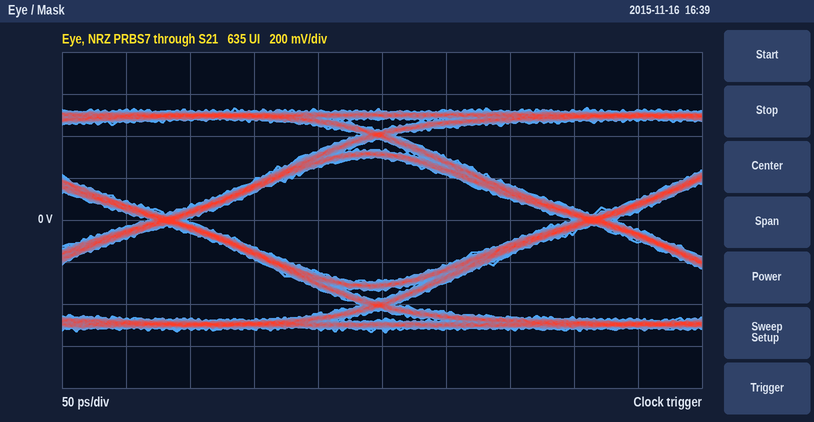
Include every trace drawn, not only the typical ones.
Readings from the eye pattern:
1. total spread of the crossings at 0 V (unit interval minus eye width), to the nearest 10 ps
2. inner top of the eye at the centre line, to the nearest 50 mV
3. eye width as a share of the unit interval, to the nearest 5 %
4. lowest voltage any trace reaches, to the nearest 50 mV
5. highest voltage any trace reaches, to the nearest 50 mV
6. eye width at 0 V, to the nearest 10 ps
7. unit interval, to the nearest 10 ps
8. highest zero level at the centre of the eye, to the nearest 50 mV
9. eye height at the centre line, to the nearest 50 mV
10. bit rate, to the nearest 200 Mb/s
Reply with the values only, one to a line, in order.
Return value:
30 ps
300 mV
90 %
-550 mV
550 mV
300 ps
330 ps
-300 mV
600 mV
3.0 Gb/s
